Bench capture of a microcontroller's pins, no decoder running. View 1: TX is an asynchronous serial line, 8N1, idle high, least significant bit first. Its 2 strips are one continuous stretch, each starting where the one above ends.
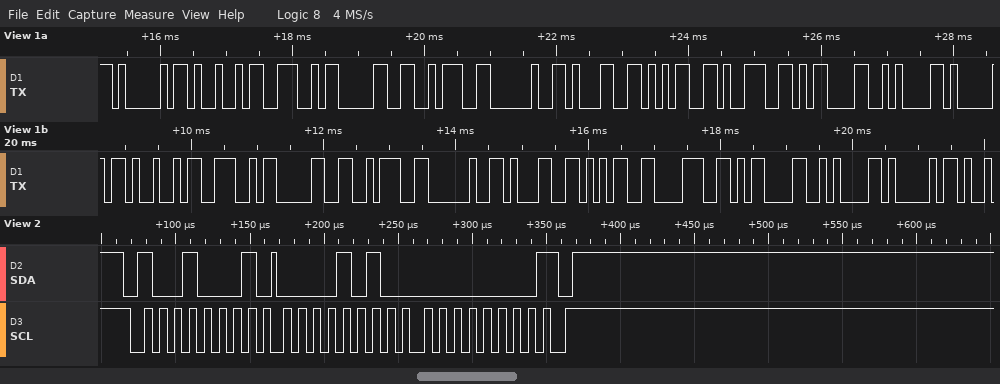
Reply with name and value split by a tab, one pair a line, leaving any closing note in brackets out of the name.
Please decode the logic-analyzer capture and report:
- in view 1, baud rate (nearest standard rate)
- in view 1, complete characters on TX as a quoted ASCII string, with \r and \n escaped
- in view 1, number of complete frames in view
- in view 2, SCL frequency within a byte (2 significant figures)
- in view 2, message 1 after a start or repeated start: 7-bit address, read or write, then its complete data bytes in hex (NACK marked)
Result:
in view 1, baud rate	9600 baud
in view 1, complete characters on TX as a quoted ASCII string, with \r and \n escaped	"AIN0: 159\r\nAIN0: 158\r\nA"
in view 1, number of complete frames in view	23
in view 2, SCL frequency within a byte	100 kHz
in view 2, message 1 after a start or repeated start: 7-bit address, read or write, then its complete data bytes in hex	0x48 read: 0A 00 NACK
